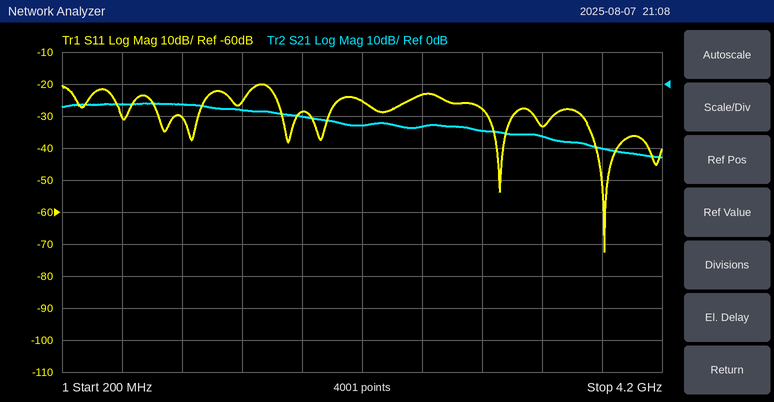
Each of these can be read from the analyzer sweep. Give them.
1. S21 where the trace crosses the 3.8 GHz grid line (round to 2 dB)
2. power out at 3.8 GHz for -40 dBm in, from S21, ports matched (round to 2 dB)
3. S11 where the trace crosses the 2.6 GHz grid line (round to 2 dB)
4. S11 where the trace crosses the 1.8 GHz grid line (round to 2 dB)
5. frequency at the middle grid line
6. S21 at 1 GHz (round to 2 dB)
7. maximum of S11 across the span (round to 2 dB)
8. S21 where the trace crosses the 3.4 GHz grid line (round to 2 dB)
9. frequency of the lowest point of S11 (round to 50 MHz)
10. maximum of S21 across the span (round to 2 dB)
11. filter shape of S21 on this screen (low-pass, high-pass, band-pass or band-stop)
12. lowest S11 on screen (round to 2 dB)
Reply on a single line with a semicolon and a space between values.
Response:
-20 dB; -60 dBm; -24 dB; -28 dB; 2.2 GHz; -6 dB; -20 dB; -16 dB; 3.80 GHz; -6 dB; low-pass; -72 dB
